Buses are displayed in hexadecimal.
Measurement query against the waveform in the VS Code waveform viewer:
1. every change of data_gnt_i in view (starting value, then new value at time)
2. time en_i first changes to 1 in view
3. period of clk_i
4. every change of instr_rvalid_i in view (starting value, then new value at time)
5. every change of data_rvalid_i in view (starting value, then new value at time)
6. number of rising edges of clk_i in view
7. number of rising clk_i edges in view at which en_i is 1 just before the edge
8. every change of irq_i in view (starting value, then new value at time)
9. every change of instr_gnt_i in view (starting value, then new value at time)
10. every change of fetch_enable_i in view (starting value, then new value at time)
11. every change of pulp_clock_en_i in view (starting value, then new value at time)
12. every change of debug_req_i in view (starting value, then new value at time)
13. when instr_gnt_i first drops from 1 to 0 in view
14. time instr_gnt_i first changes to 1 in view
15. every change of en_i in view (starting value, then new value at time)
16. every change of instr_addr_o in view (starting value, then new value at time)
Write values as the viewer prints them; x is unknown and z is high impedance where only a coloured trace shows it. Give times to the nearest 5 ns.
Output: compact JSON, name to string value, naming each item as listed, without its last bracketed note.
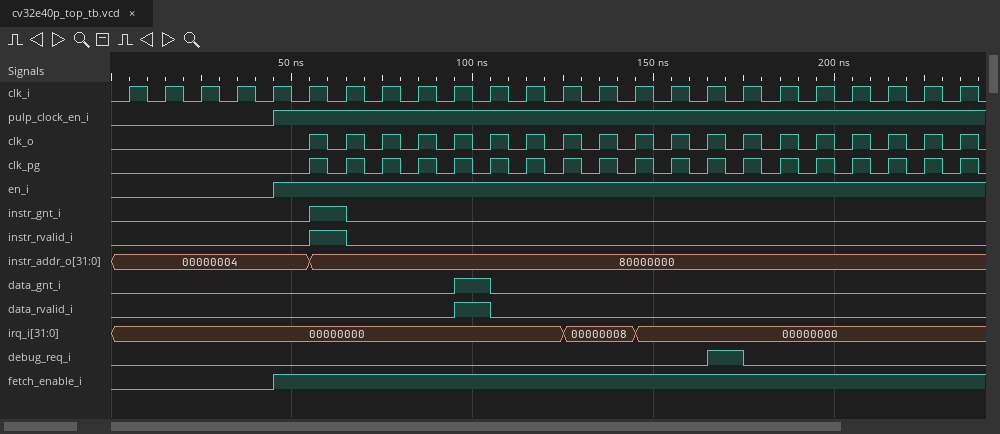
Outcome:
{"every change of data_gnt_i in view": "0, 1 at 95 ns, 0 at 105 ns", "time en_i first changes to 1 in view": "45 ns", "period of clk_i": "10 ns", "every change of instr_rvalid_i in view": "0, 1 at 55 ns, 0 at 65 ns", "every change of data_rvalid_i in view": "0, 1 at 95 ns, 0 at 105 ns", "number of rising edges of clk_i in view": "24", "number of rising clk_i edges in view at which en_i is 1 just before the edge": "19", "every change of irq_i in view": "00000000, 00000008 at 125 ns, 00000000 at 145 ns", "every change of instr_gnt_i in view": "0, 1 at 55 ns, 0 at 65 ns", "every change of fetch_enable_i in view": "0, 1 at 45 ns", "every change of pulp_clock_en_i in view": "0, 1 at 45 ns", "every change of debug_req_i in view": "0, 1 at 165 ns, 0 at 175 ns", "when instr_gnt_i first drops from 1 to 0 in view": "65 ns", "time instr_gnt_i first changes to 1 in view": "55 ns", "every change of en_i in view": "0, 1 at 45 ns", "every change of instr_addr_o in view": "00000004, 80000000 at 55 ns"}
